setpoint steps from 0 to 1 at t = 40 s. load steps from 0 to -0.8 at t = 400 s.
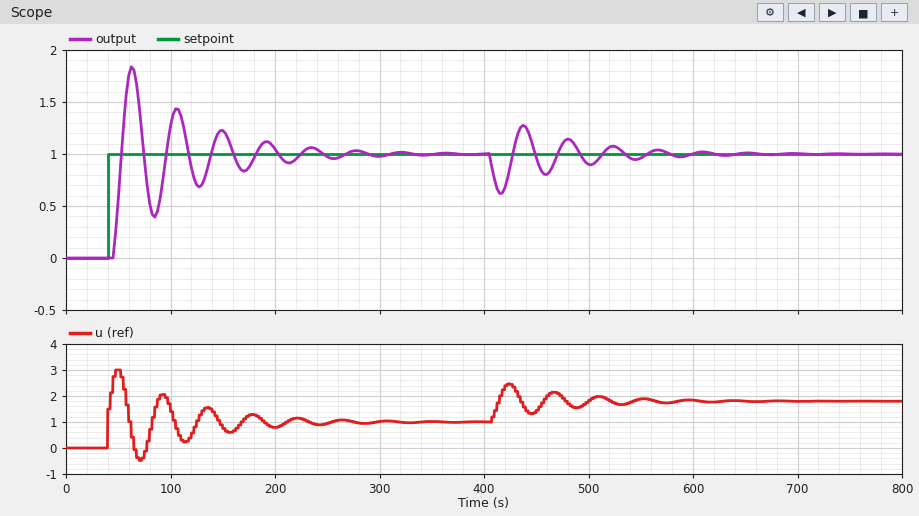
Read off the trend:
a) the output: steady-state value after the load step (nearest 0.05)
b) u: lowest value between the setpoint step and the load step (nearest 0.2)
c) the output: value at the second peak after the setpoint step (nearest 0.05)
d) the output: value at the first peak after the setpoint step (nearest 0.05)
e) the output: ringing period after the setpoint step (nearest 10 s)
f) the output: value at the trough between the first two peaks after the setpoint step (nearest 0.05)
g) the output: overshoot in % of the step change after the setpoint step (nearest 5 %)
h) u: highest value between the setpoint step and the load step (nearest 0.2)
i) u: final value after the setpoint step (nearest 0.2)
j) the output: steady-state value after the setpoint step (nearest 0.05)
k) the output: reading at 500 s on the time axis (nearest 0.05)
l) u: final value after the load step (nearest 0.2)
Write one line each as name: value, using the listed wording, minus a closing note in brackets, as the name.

the output: steady-state value after the load step: 1.00
u: lowest value between the setpoint step and the load step: -0.4
the output: value at the second peak after the setpoint step: 1.45
the output: value at the first peak after the setpoint step: 1.85
the output: ringing period after the setpoint step: 40 s
the output: value at the trough between the first two peaks after the setpoint step: 0.40
the output: overshoot in % of the step change after the setpoint step: 85 %
u: highest value between the setpoint step and the load step: 3.0
u: final value after the setpoint step: 1.0
the output: steady-state value after the setpoint step: 1.00
the output: reading at 500 s on the time axis: 0.90
u: final value after the load step: 1.8
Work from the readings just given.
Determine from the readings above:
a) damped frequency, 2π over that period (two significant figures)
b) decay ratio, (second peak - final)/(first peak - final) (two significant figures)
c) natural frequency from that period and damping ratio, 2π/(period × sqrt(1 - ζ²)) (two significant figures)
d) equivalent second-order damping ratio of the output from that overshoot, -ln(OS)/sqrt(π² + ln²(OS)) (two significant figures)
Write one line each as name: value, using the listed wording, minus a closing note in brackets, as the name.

damped frequency, 2π over that period: 0.16 rad/s
decay ratio, (second peak - final)/(first peak - final): 0.53
natural frequency from that period and damping ratio, 2π/(period × sqrt(1 - ζ²)): 0.16 rad/s
equivalent second-order damping ratio of the output from that overshoot, -ln(OS)/sqrt(π² + ln²(OS)): 0.052
